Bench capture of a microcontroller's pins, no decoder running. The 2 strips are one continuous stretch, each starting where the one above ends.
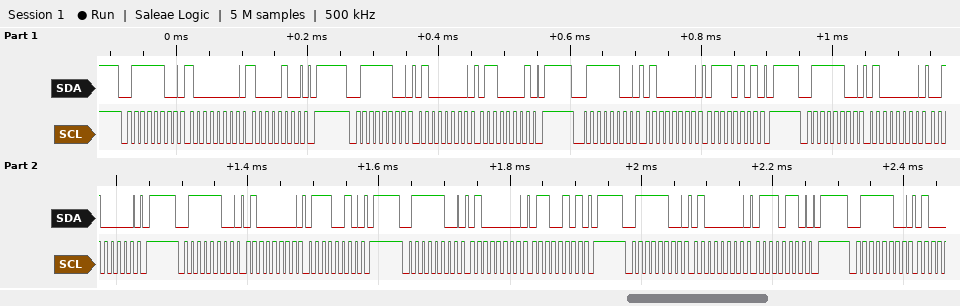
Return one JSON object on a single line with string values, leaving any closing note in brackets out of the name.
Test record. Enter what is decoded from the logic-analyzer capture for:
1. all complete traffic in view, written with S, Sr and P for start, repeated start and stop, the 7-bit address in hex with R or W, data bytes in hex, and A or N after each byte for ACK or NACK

{"all complete traffic in view, written with S, Sr and P for start, repeated start and stop, the 7-bit address in hex with R or W, data bytes in hex, and A or N after each byte for ACK or NACK": "S 3EW A 80 A 84 A P S 3EW A 40 A 61 A P S 3EW A 40 A 75 A P S 3EW A 40 A 20 A P S 3EW A 40 A 72 A P S 3EW A 40 A 65 A P S 3EW A 40 A 76 A P S 3EW A"}
